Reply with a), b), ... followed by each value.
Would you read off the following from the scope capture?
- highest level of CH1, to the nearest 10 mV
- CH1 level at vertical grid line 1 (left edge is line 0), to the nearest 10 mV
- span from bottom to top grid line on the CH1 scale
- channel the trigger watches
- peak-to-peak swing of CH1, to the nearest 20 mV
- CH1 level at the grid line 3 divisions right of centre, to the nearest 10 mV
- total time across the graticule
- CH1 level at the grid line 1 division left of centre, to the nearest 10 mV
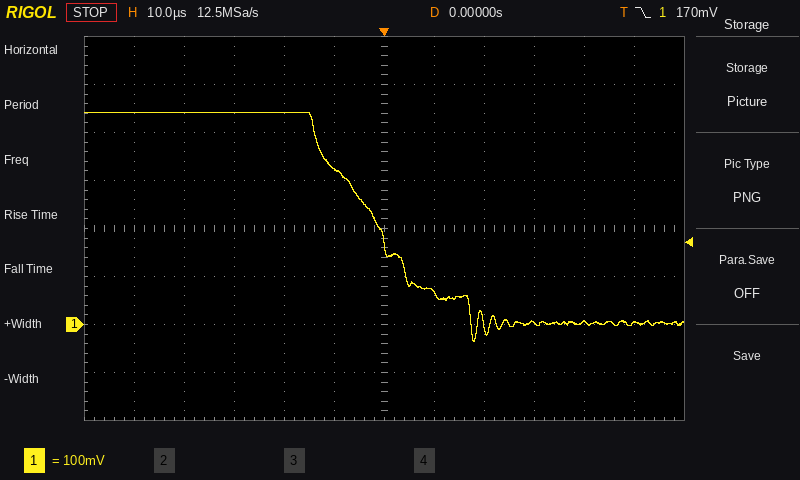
a) 440 mV
b) 440 mV
c) 800 mV
d) CH1
e) 480 mV
f) 0 mV
g) 120 µs
h) 320 mV
